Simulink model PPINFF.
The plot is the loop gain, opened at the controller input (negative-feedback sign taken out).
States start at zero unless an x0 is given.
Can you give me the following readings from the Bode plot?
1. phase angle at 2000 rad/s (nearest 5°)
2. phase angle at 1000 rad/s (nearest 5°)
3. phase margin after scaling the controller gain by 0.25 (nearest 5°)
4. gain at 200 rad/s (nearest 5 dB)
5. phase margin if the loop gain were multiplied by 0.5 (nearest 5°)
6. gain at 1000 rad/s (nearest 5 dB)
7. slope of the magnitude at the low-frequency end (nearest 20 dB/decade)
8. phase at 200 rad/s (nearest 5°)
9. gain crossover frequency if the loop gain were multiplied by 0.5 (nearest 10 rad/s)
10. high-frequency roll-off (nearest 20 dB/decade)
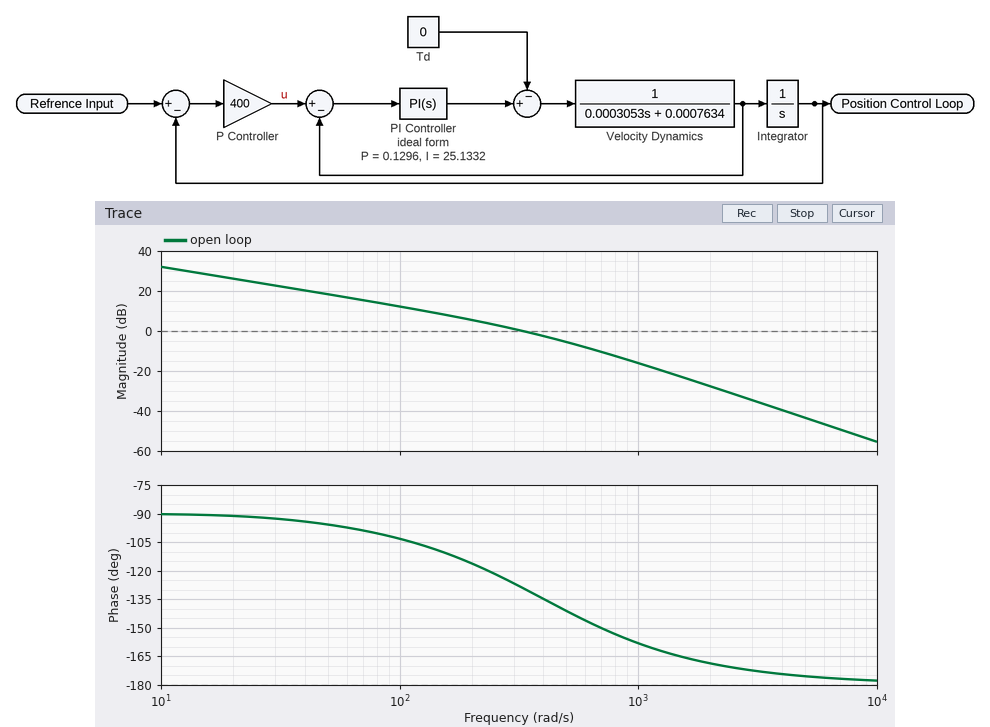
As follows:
-170°
-160°
75°
5 dB
65°
-15 dB
-20 dB/decade
-115°
190 rad/s
-40 dB/decade
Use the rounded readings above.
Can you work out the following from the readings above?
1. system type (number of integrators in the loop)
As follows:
1
